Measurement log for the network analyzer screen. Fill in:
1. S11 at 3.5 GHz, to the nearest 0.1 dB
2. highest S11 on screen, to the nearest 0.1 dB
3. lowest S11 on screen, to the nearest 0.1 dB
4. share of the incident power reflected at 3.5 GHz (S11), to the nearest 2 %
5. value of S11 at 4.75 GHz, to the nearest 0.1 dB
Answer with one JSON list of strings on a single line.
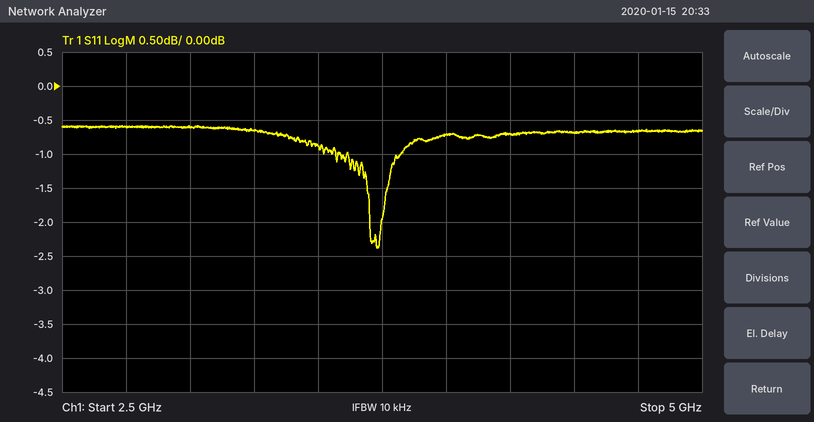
["-0.9 dB", "-0.6 dB", "-2.4 dB", "82 %", "-0.7 dB"]
